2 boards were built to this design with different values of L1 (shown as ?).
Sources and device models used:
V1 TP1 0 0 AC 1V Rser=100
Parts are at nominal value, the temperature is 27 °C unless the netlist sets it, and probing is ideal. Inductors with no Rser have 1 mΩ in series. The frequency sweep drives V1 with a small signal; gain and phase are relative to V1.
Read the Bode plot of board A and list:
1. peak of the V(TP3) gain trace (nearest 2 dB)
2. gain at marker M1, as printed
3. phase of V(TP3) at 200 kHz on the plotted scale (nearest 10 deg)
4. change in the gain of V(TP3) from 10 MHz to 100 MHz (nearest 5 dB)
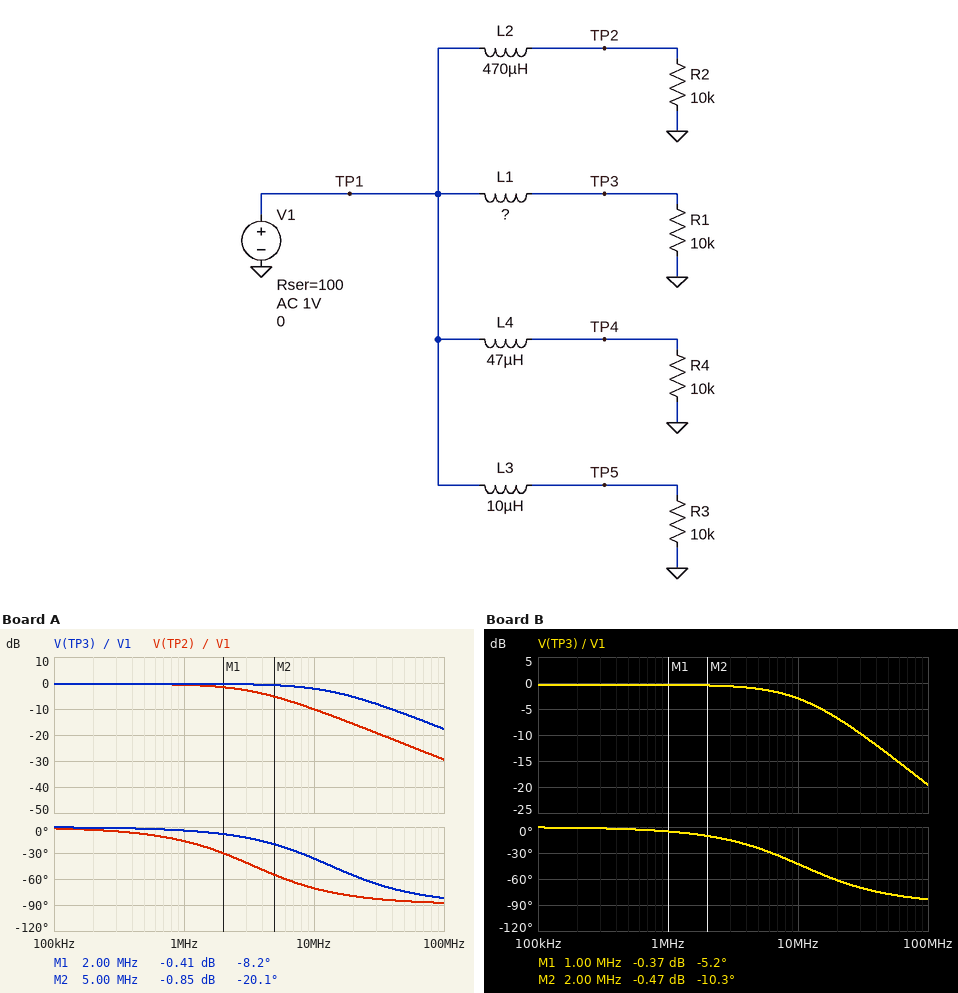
0 dB
-0.41 dB
0 deg
-15 dB
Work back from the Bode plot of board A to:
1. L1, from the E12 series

120 µH
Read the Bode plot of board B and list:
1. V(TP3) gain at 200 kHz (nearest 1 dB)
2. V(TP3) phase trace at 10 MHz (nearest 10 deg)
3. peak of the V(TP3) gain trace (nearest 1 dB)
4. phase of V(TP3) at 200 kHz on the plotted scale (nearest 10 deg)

0 dB
-40 deg
0 dB
0 deg
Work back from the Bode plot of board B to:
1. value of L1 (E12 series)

150 µH
